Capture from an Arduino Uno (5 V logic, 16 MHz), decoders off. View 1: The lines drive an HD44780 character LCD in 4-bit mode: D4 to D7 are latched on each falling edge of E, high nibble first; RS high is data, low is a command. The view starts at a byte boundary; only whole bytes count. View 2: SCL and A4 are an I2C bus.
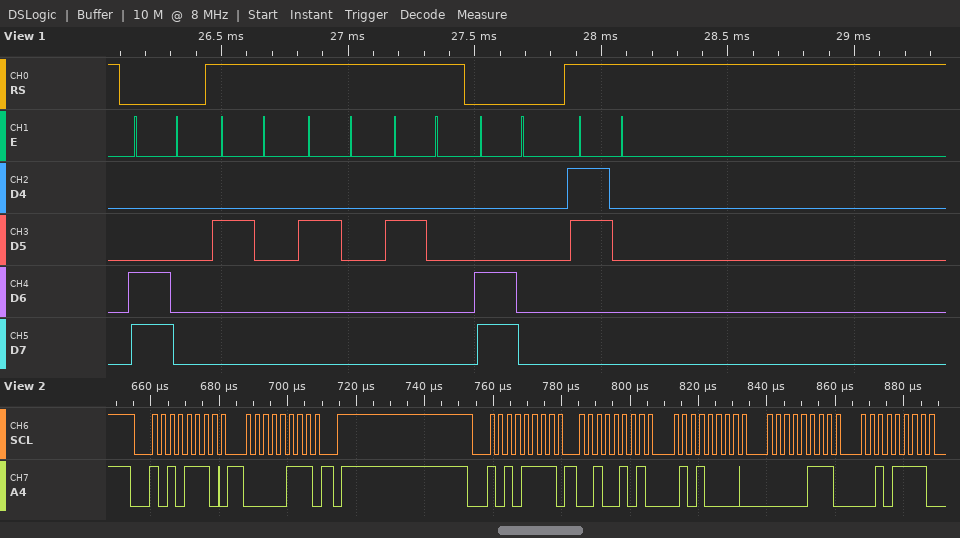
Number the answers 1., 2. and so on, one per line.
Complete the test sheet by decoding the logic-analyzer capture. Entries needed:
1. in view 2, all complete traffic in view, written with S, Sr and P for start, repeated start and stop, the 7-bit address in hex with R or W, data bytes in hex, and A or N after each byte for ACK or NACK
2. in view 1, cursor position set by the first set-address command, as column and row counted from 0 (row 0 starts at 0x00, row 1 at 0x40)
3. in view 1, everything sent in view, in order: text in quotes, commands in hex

1. S 57W A 07 A P S 57R A 25 A 50 A 07 A 2F A
2. column 0, row 1
3. 0xC0 "   " 0xC0 "0"
